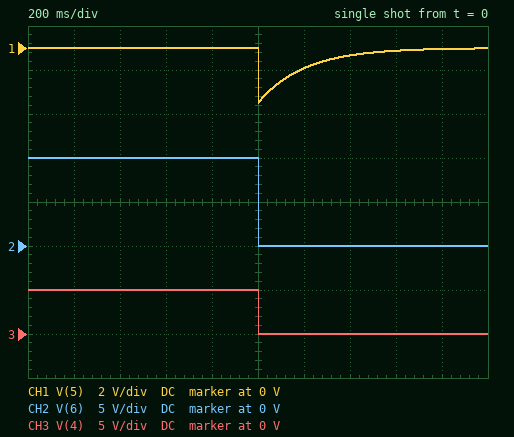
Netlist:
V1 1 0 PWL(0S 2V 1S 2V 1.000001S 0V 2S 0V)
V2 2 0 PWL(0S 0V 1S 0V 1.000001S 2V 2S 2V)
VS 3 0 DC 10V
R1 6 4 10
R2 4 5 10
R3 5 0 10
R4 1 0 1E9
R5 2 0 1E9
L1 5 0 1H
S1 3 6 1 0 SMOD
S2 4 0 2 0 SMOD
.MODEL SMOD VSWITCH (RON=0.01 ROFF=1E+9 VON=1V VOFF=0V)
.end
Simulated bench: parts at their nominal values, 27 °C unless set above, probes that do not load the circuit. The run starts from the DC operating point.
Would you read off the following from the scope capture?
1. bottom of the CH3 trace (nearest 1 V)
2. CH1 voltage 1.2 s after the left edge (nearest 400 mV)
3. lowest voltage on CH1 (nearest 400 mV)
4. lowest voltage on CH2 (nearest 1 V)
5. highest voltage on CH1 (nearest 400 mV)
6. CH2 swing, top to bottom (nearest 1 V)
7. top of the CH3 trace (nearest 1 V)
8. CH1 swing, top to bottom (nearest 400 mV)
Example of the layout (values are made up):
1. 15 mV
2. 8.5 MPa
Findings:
1. 0 V
2. -800 mV
3. -2.4 V
4. 0 V
5. 0 V
6. 10 V
7. 5 V
8. 2.4 V
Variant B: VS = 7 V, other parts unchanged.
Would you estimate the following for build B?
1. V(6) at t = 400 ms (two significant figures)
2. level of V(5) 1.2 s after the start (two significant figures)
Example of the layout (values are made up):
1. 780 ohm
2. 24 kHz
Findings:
1. 7.0 V
2. -640 mV
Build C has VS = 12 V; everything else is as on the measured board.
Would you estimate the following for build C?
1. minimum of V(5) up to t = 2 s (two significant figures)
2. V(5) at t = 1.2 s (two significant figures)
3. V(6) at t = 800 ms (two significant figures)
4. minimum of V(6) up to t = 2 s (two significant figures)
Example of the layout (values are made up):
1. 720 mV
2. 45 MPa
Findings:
1. -3.0 V
2. -1.1 V
3. 12 V
4. -3.0 mV
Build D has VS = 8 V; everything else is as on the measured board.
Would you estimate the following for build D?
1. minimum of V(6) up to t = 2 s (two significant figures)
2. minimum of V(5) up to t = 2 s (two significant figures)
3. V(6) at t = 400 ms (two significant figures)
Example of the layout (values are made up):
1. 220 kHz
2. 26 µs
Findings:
1. -2.0 mV
2. -2.0 V
3. 8.0 V
